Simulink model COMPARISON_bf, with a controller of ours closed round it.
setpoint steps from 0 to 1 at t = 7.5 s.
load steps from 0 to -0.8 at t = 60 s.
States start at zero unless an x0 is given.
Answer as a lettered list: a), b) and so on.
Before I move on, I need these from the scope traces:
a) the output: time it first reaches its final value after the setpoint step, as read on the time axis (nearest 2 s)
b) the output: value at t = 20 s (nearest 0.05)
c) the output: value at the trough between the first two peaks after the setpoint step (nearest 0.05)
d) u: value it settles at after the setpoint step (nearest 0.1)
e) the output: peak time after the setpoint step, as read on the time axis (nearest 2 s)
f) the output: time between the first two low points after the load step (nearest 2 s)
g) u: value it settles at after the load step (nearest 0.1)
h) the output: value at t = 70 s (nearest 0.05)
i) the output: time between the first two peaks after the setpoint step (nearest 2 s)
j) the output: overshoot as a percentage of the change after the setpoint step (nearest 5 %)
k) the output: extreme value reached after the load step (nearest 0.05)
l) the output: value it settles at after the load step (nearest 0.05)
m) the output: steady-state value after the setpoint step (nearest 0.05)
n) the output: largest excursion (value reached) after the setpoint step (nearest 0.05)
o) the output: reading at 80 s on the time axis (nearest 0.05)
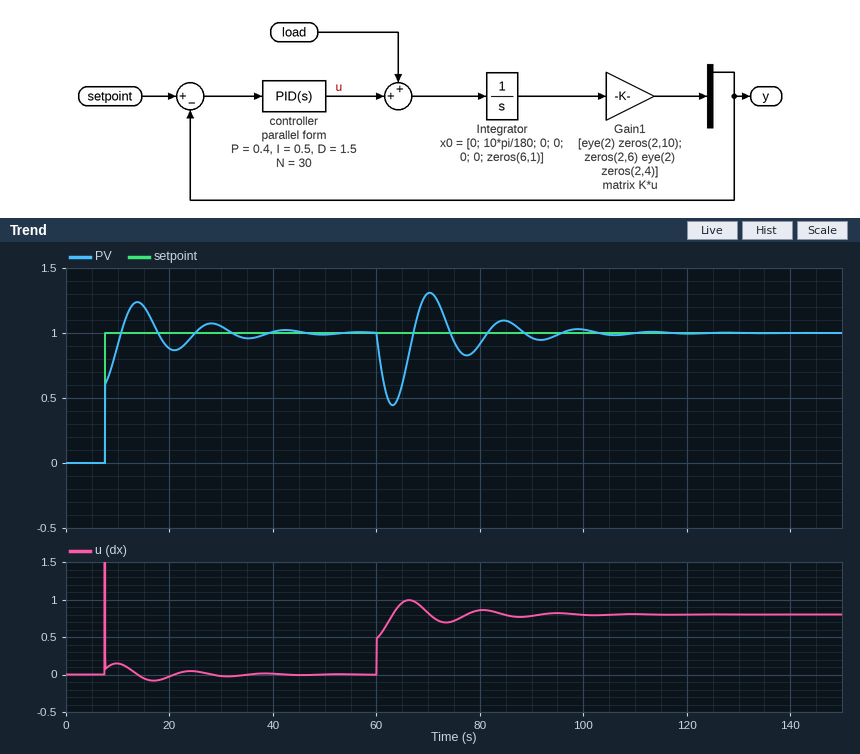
a) 10 s
b) 0.90
c) 0.85
d) 0.0
e) 14 s
f) 14 s
g) 0.8
h) 1.30
i) 14 s
j) 25 %
k) 0.45
l) 1.00
m) 1.00
n) 1.25
o) 0.90
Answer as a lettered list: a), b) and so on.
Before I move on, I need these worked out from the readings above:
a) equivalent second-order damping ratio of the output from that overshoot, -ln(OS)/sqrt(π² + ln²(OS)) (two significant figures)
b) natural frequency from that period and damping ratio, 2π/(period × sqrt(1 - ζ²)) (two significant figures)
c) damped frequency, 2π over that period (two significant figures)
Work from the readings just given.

a) 0.40
b) 0.49 rad/s
c) 0.45 rad/s
